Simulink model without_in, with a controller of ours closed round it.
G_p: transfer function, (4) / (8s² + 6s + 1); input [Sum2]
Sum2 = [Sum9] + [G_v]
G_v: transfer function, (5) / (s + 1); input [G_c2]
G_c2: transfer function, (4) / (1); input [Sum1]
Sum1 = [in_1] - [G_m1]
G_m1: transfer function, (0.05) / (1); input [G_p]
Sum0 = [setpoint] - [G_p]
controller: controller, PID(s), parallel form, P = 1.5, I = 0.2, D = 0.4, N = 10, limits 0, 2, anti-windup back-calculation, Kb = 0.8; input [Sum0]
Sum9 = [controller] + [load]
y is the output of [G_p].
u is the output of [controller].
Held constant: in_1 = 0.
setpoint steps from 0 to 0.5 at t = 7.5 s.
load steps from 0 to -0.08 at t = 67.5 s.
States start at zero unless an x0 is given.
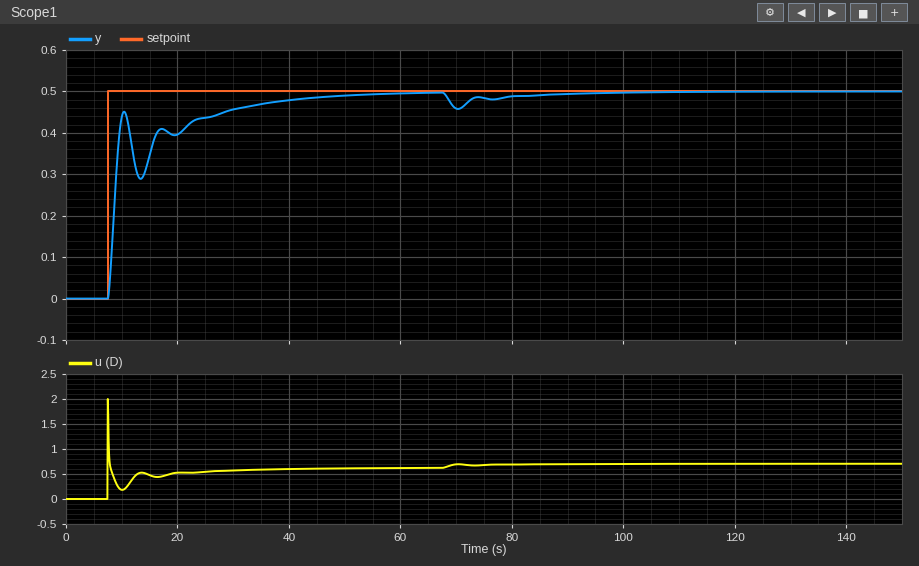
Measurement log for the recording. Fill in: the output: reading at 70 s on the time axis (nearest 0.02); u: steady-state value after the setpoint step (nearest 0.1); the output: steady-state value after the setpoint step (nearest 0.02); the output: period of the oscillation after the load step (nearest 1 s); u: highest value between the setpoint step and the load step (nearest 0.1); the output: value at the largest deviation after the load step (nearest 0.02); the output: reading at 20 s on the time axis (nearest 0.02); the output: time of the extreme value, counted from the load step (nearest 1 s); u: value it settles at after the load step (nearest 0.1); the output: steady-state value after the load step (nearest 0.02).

0.46
0.6
0.50
6 s
2.0
0.46
0.40
3 s
0.7
0.50
